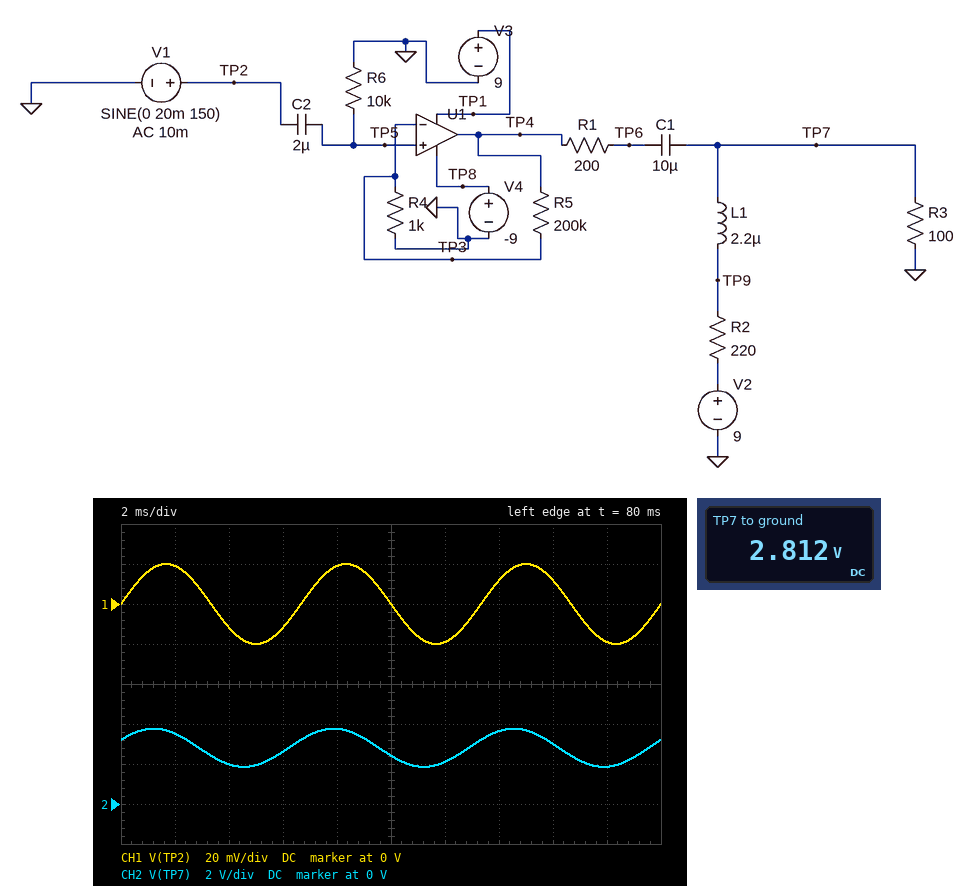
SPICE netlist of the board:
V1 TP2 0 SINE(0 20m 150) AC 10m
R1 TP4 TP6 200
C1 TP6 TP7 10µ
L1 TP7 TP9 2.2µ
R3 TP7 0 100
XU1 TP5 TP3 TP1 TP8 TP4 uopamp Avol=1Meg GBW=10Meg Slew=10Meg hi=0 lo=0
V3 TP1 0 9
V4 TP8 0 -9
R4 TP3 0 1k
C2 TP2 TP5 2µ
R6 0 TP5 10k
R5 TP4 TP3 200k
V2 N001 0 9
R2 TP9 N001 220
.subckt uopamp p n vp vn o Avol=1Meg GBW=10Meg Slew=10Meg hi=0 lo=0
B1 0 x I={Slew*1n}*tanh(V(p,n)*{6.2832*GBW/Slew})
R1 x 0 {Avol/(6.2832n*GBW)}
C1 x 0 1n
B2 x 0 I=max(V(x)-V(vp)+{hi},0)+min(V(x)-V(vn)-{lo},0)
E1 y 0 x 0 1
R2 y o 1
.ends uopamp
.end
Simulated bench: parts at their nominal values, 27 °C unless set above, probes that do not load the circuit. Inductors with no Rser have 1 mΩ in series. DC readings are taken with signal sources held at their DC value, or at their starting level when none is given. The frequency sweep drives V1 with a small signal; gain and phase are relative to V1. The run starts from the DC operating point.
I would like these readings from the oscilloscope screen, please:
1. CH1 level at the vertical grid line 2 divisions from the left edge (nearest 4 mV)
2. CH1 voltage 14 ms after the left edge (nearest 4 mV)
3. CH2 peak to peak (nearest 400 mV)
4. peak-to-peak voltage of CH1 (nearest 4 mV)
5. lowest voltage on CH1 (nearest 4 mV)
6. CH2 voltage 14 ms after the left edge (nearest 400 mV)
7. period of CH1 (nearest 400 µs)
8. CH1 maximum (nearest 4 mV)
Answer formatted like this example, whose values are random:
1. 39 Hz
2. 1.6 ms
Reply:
1. -12 mV
2. 12 mV
3. 2.0 V
4. 40 mV
5. -20 mV
6. 3.6 V
7. 6.8 ms
8. 20 mV
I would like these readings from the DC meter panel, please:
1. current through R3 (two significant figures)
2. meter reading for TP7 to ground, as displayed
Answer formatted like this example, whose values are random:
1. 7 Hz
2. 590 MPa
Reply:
1. 28 mA
2. 2.812 V
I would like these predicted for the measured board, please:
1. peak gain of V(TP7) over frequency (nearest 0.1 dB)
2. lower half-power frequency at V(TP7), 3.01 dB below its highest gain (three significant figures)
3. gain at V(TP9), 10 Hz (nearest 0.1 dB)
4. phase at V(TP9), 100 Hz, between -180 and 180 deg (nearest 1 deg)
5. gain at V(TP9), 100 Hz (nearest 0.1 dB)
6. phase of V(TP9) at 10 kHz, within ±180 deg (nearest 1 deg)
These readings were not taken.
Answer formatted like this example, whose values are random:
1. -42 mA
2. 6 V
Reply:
1. 34.2 dB
2. 60.1 Hz
3. 16.5 dB
4. 35 deg
5. 32.9 dB
6. -11 deg
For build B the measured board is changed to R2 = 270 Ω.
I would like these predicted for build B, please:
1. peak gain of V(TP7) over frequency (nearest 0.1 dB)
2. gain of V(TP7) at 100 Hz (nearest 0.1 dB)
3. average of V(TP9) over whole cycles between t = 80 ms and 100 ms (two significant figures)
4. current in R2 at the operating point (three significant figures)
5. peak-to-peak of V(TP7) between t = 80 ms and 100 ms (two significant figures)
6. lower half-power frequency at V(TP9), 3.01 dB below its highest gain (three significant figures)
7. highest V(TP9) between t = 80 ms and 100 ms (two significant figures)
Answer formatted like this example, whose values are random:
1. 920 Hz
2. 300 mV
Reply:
1. 34.6 dB
2. 33.3 dB
3. 2.4 V
4. 24.3 mA
5. 2.0 V
6. 59.2 Hz
7. 3.4 V
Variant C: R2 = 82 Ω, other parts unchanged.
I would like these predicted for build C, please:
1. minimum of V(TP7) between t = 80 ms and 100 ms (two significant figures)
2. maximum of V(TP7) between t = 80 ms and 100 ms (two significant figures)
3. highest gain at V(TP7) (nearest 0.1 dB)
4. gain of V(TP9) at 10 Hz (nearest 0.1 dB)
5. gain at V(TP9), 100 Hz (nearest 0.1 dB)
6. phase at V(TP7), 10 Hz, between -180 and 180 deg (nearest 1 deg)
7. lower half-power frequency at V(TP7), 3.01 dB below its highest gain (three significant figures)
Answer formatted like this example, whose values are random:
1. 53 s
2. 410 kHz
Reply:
1. 4.3 V
2. 5.6 V
3. 31.3 dB
4. 12.9 dB
5. 29.8 dB
6. 120 deg
7. 65.7 Hz
